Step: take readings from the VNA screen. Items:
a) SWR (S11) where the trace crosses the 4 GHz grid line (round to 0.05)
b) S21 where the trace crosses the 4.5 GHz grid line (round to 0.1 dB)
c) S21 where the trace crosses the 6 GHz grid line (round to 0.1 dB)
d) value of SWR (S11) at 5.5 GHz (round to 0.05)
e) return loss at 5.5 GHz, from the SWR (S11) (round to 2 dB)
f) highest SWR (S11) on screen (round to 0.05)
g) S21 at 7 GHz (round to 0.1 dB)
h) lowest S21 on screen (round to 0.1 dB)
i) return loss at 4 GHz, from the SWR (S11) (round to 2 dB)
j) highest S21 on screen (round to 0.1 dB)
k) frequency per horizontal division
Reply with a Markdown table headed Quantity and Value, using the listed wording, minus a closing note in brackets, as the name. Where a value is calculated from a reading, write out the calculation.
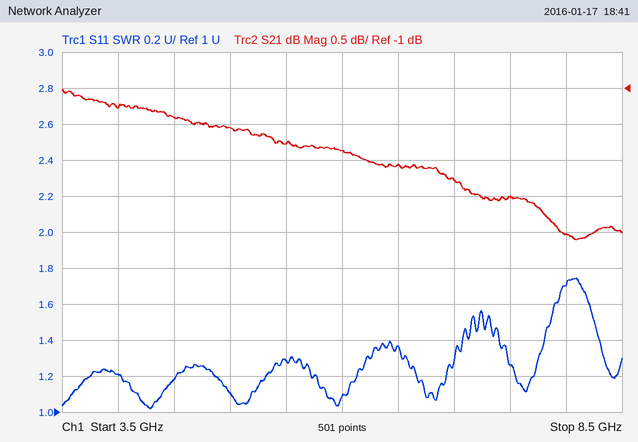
| Quantity | Value |
|---|---|
| SWR (S11) where the trace crosses the 4 GHz grid line | 1.20 |
| S21 where the trace crosses the 4.5 GHz grid line | -1.4 dB |
| S21 where the trace crosses the 6 GHz grid line | -1.9 dB |
| value of SWR (S11) at 5.5 GHz | 1.30 |
| return loss at 5.5 GHz, from the SWR (S11) | −20 log10((1.3 − 1)/(1.3 + 1)) ≈ 18 dB |
| highest SWR (S11) on screen | 1.75 |
| S21 at 7 GHz | -2.3 dB |
| lowest S21 on screen | -3.1 dB |
| return loss at 4 GHz, from the SWR (S11) | −20 log10((1.2 − 1)/(1.2 + 1)) ≈ 20.8 dB, so 20 dB to the nearest 2 dB |
| highest S21 on screen | -1.0 dB |
| frequency per horizontal division | 500 MHz |
